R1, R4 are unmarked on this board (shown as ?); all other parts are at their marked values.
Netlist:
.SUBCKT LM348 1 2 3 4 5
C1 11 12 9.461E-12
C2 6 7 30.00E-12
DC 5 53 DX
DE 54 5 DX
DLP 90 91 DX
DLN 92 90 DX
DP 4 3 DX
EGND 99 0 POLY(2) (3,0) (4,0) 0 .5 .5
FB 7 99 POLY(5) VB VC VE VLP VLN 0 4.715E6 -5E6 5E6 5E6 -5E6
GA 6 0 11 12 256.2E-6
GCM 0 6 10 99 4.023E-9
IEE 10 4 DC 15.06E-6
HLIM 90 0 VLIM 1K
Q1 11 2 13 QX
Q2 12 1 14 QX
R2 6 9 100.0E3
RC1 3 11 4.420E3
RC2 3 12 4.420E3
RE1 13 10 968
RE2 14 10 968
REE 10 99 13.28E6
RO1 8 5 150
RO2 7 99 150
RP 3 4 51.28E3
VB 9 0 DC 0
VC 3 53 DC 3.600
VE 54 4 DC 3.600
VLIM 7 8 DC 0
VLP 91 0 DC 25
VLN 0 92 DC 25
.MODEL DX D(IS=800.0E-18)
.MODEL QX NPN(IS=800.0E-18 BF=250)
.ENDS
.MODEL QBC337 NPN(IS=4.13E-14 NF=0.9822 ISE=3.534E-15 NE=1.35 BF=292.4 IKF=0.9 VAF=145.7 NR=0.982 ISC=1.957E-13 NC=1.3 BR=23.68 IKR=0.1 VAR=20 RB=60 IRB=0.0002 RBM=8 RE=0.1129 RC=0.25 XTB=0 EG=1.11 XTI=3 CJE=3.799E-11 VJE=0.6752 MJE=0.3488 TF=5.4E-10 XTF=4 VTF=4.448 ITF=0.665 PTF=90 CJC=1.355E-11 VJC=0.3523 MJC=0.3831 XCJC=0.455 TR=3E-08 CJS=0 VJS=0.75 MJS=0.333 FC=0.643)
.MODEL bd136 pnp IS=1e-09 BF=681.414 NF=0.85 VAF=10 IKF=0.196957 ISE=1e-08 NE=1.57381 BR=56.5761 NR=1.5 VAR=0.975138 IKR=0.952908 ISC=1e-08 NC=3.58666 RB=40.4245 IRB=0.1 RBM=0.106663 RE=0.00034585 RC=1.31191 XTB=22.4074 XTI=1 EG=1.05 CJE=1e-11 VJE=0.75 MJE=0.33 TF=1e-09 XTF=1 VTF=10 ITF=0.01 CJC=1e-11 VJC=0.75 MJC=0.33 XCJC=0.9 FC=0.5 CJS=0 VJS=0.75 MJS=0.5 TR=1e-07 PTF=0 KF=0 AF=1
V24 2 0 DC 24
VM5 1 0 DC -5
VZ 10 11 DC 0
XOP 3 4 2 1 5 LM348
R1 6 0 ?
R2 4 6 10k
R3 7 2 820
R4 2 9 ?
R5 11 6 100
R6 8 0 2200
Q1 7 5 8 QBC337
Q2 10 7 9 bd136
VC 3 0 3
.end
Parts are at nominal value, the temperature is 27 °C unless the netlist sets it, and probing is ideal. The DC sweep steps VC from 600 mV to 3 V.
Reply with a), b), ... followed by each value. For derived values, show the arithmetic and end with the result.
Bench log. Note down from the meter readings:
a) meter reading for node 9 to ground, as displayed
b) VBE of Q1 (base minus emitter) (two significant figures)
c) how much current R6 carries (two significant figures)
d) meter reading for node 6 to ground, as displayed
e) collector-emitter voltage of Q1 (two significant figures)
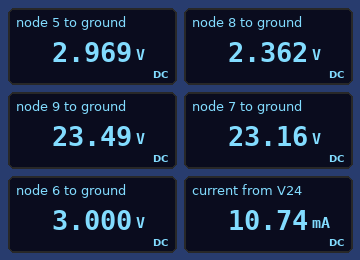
a) 23.49 V
b) 2.969 V - 2.362 V = 610 mV
c) (2.362 V) / 2.2 kΩ = 1.1 mA
d) 3.000 V
e) 23.16 V - 2.362 V = 21 V
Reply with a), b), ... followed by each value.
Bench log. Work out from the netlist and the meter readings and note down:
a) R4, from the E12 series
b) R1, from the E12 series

a) 56 Ω
b) 330 Ω
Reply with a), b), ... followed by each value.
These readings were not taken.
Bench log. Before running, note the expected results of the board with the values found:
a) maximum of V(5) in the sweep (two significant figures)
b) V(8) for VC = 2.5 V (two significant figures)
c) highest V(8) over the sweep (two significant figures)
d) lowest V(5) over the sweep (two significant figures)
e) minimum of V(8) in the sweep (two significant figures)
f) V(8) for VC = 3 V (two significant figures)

a) 3.0 V
b) 2.1 V
c) 2.4 V
d) 1.7 V
e) 1.1 V
f) 2.4 V
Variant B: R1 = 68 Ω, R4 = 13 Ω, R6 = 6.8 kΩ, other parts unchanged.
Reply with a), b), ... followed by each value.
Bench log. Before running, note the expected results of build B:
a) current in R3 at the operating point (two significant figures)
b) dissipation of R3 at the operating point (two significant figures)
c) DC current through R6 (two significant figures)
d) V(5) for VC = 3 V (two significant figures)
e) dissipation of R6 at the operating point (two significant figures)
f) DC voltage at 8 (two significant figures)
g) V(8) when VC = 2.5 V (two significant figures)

a) 1.2 mA
b) 1.1 mW
c) 1.3 mA
d) 9.4 V
e) 11 mW
f) 8.8 V
g) 7.8 V
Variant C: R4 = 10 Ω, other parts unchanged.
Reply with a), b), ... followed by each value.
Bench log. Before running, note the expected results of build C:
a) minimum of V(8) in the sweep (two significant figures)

a) 870 mV
